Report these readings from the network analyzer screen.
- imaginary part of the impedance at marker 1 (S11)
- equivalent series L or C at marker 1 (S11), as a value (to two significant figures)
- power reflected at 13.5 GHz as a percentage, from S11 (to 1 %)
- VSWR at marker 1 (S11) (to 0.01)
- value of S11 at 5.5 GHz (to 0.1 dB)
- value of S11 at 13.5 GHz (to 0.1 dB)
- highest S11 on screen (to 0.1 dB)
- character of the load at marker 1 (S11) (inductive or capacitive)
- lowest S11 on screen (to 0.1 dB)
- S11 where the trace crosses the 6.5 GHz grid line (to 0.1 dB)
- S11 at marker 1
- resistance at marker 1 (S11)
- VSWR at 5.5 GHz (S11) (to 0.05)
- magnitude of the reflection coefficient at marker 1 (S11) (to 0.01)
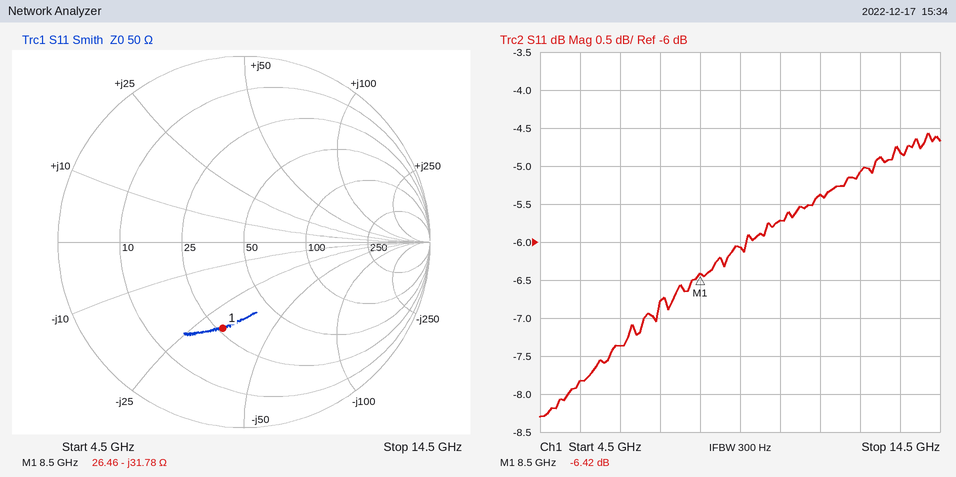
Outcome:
-31.78 Ω
590 fF
33 %
2.83
-7.8 dB
-4.8 dB
-4.6 dB
capacitive
-8.3 dB
-7.4 dB
-6.42 dB
26.46 Ω
2.35
0.48
